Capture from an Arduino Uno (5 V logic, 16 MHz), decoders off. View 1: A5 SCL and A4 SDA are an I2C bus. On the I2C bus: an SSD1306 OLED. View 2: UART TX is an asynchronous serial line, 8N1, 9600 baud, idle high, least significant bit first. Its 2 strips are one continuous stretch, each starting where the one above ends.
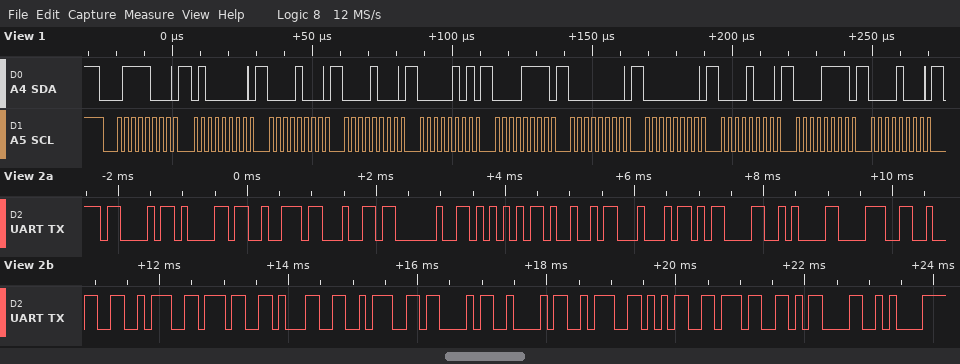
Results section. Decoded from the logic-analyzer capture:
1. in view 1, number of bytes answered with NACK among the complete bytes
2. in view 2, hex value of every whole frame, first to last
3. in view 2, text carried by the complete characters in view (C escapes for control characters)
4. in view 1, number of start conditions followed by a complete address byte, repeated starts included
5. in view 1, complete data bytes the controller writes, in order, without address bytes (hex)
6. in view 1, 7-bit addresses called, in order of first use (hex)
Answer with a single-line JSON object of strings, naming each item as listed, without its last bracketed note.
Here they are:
{"in view 1, number of bytes answered with NACK among the complete bytes": "0", "in view 2, hex value of every whole frame, first to last": "0x43 0x61 0x72 0x64 0x20 0x55 0x49 0x44 0x0D 0x0A 0x38 0x32 0x3A 0x37 0x31 0x3A 0x43 0x42 0x3A 0x35 0x37 0x0D 0x0A", "in view 2, text carried by the complete characters in view": "\"Card UID\\r\\n82:71:CB:57\\r\\n\"", "in view 1, number of start conditions followed by a complete address byte, repeated starts included": "1", "in view 1, complete data bytes the controller writes, in order, without address bytes": "40 08 08 05 0F 00 00 08 0F 08", "in view 1, 7-bit addresses called, in order of first use": "0x3C"}
